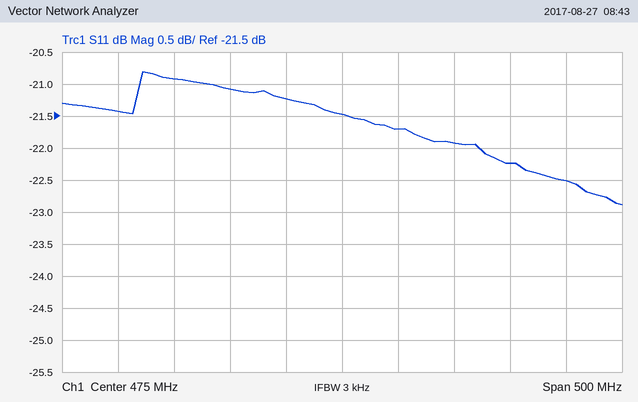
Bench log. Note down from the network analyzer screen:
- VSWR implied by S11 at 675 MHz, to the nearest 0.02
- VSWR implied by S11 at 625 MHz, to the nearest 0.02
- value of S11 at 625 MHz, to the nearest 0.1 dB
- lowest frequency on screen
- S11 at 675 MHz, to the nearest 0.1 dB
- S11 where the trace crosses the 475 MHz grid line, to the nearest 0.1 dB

1.16
1.16
-22.2 dB
225 MHz
-22.5 dB
-21.5 dB
